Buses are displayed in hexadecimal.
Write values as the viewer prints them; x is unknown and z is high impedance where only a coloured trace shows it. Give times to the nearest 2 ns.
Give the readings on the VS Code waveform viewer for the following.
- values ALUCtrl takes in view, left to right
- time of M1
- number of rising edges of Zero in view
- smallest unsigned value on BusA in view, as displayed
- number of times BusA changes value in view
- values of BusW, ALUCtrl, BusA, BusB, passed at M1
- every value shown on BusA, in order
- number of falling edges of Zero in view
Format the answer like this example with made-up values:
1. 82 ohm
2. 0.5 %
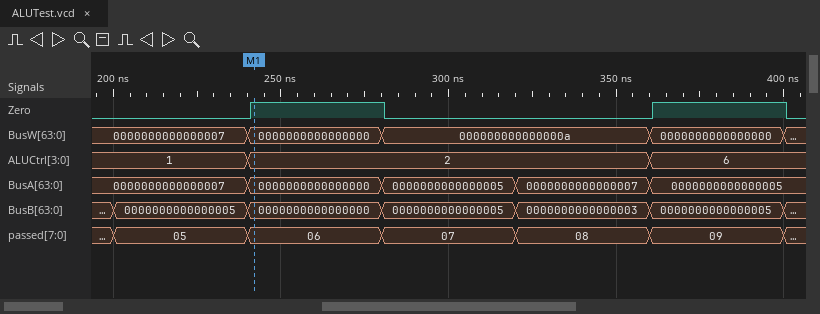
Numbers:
1. 1, 2, 6
2. 242 ns
3. 2
4. 0000000000000000
5. 4
6. BusW=0000000000000000, ALUCtrl=2, BusA=0000000000000000, BusB=0000000000000000, passed=06
7. 0000000000000007, 0000000000000000, 0000000000000005, 0000000000000007, 0000000000000005
8. 2
